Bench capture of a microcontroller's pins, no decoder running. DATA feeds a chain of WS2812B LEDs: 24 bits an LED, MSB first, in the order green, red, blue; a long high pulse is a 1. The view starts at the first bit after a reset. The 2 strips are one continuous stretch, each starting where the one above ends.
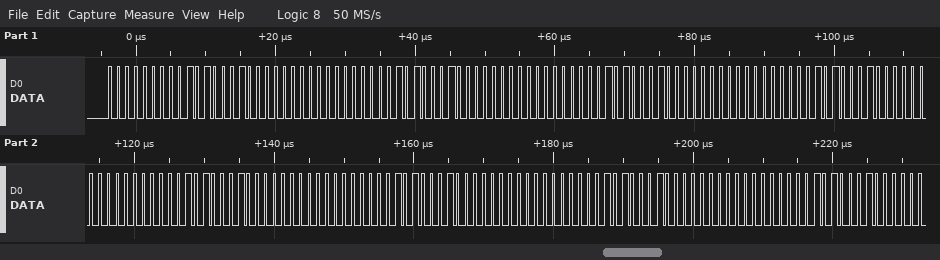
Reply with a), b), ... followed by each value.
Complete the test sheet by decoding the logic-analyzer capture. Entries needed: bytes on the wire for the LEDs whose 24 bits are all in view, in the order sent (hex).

a) 00 51 00 00 51 00 00 51 00 00 51 00 00 51 00 00 51 00 00 51 00
